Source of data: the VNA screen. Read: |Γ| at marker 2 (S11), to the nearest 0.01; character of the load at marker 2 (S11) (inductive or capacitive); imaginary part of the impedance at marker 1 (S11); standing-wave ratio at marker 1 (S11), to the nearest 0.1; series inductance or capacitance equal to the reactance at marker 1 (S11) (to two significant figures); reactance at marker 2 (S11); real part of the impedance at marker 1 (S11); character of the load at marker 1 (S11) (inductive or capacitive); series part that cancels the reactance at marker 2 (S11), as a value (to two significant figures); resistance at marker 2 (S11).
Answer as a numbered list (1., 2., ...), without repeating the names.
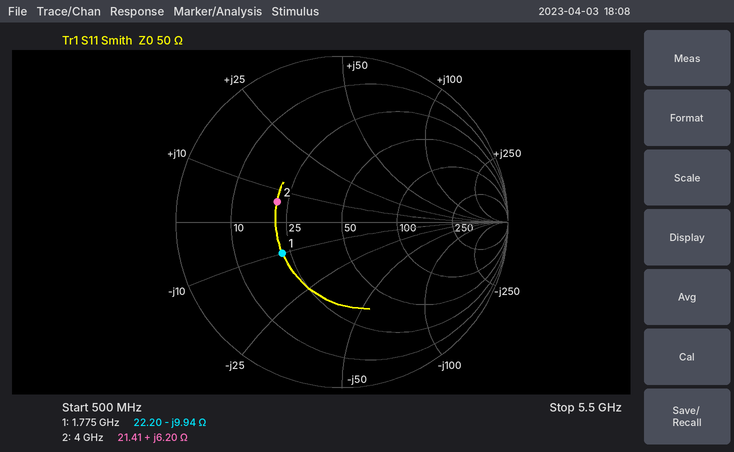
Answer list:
1. 0.41
2. inductive
3. -9.94 Ω
4. 2.4
5. 9.0 pF
6. +6.20 Ω
7. 22.20 Ω
8. capacitive
9. 6.4 pF
10. 21.41 Ω
